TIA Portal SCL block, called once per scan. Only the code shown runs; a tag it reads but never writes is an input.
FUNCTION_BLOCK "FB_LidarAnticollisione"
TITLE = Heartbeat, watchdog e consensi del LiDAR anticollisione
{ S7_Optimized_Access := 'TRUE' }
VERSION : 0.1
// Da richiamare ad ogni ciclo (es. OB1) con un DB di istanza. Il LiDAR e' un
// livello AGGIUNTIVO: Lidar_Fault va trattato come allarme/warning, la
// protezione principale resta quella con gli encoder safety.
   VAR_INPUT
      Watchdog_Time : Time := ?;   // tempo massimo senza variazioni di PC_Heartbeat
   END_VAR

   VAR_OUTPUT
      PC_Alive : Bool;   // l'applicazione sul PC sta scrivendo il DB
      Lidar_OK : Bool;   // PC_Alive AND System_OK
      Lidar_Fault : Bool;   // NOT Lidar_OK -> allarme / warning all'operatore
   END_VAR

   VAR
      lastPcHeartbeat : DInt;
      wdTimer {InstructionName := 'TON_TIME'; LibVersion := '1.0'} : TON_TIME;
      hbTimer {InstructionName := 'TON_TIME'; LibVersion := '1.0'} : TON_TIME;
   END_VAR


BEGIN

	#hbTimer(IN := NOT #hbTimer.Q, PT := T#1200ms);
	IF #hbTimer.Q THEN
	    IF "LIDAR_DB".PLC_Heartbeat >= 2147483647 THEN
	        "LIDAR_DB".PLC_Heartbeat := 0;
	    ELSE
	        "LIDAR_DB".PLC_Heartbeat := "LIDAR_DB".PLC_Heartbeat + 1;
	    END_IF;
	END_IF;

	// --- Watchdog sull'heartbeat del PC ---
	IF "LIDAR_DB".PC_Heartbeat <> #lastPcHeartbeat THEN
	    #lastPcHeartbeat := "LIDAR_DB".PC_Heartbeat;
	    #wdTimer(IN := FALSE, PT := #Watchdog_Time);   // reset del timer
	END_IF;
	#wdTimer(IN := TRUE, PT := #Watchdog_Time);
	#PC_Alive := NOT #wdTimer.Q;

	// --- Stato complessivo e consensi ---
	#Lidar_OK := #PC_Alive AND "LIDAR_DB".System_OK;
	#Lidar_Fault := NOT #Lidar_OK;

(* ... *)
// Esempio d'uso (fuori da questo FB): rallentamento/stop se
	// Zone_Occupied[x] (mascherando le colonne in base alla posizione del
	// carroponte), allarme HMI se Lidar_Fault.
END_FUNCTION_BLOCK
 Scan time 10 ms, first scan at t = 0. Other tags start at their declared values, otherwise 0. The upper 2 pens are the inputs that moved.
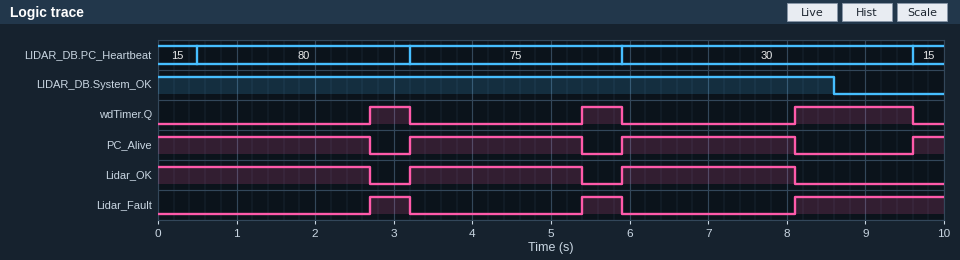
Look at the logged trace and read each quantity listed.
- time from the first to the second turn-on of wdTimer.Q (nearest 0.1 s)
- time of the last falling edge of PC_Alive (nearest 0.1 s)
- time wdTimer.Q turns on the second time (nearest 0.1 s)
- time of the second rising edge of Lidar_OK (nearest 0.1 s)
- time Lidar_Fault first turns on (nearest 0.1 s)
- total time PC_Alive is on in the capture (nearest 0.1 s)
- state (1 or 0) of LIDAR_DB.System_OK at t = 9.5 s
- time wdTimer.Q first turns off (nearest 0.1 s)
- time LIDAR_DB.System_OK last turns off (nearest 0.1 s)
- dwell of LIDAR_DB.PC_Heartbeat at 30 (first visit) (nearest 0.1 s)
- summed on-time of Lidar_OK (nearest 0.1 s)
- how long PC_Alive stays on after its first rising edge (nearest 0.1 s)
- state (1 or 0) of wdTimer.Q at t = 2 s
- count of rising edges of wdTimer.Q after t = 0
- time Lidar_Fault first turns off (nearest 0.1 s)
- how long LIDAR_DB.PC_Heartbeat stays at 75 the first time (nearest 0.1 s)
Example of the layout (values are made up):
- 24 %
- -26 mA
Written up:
- 2.7 s
- 8.1 s
- 5.4 s
- 5.9 s
- 2.7 s
- 7.5 s
- 0
- 3.2 s
- 8.6 s
- 3.7 s
- 7.1 s
- 2.2 s
- 0
- 3
- 3.2 s
- 2.7 s
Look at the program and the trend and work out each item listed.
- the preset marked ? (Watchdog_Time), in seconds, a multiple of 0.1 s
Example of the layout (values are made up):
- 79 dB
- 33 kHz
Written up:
- 2.2 s
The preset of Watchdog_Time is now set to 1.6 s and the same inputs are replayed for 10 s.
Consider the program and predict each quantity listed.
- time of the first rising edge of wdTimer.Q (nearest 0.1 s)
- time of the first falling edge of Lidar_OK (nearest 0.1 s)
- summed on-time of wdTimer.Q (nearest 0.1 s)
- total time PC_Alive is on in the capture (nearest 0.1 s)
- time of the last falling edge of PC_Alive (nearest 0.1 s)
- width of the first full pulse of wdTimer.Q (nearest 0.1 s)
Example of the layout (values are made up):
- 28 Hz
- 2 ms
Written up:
- 2.1 s
- 2.1 s
- 4.3 s
- 5.7 s
- 7.5 s
- 1.1 s
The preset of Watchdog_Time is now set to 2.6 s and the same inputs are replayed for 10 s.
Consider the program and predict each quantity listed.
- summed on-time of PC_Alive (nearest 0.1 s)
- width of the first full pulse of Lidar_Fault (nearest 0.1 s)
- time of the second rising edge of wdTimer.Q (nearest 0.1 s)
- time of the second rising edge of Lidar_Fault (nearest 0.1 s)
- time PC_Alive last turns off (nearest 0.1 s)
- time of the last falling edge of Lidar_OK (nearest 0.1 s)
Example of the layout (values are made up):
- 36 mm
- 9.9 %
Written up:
- 8.7 s
- 0.1 s
- 5.8 s
- 5.8 s
- 8.5 s
- 8.5 s
